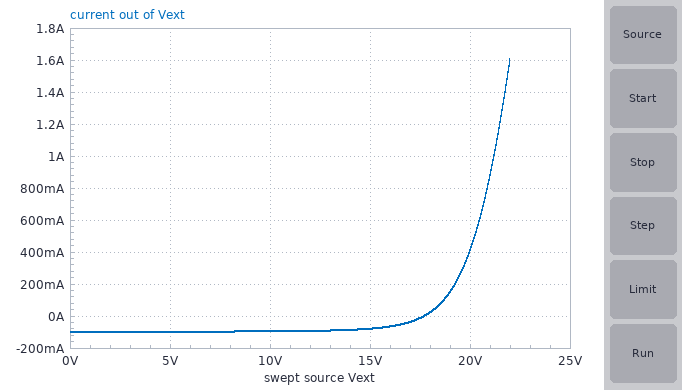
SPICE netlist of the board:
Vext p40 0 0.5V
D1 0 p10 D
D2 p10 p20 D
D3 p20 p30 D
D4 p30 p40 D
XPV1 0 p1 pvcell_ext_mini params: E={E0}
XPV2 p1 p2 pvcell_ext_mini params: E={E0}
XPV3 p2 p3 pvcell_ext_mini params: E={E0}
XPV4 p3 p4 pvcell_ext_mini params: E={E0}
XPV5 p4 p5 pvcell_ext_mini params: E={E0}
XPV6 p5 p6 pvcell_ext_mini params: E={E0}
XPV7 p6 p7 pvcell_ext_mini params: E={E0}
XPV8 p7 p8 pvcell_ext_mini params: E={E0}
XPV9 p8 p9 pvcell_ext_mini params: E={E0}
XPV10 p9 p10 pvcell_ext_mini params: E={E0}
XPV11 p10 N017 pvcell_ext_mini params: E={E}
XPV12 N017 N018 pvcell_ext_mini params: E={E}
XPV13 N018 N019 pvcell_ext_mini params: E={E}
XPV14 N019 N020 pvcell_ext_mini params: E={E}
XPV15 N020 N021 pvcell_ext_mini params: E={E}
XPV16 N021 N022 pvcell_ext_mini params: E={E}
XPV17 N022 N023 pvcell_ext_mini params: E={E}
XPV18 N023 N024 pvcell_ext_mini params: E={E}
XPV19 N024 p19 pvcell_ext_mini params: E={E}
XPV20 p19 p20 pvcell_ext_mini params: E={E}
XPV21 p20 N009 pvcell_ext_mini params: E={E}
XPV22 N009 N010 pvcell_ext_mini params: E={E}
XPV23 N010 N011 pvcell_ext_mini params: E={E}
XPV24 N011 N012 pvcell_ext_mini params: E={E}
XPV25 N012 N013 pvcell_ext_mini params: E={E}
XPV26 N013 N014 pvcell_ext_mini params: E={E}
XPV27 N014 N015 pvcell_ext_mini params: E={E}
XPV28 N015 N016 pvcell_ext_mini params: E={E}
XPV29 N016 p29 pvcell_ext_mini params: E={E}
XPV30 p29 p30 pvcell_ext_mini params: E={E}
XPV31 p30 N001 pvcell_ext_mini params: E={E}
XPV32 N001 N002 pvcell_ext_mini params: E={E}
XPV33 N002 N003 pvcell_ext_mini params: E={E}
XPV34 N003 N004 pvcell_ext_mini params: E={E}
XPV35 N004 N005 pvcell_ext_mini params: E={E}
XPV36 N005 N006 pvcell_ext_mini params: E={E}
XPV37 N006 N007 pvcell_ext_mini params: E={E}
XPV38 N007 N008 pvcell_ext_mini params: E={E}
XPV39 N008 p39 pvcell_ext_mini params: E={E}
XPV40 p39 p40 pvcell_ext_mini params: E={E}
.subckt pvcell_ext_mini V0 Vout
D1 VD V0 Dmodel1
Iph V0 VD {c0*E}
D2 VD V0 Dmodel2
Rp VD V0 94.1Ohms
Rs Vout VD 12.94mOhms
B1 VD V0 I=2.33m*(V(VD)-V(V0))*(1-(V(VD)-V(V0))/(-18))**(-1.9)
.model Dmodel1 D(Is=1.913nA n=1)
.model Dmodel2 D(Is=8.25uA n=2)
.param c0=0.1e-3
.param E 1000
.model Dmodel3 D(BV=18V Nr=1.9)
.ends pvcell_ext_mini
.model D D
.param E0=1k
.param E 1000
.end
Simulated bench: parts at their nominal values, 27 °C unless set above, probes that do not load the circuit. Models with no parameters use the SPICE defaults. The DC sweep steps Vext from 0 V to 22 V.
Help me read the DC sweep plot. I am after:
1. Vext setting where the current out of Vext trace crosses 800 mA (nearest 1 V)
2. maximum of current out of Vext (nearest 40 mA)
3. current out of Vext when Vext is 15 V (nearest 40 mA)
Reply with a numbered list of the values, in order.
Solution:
1. 21 V
2. 1.60 A
3. -80 mA
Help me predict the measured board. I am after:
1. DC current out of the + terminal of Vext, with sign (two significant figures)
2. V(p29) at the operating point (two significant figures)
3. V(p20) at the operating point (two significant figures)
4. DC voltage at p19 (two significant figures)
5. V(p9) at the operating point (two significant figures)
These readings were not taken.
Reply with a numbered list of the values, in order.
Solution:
1. -100 mA
2. 360 mV
3. 250 mV
4. 240 mV
5. 110 mV
